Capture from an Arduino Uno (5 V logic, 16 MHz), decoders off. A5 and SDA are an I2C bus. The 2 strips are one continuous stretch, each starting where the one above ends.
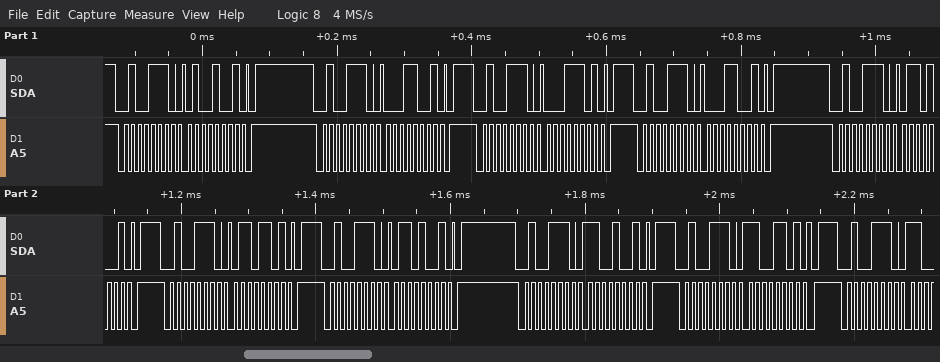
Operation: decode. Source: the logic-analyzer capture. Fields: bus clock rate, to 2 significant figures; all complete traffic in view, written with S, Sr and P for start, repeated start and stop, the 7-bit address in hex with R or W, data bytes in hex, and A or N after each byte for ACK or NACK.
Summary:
100 kHz
S 27W A 49 A P S 27W A 19 A P S 27W A 1D A P S 27W A 19 A P S 27W A 69 A P S 27W A 6D A P S 27W A 69 A P S 27W A C9 A P S 27W A CD A P S 27W A
